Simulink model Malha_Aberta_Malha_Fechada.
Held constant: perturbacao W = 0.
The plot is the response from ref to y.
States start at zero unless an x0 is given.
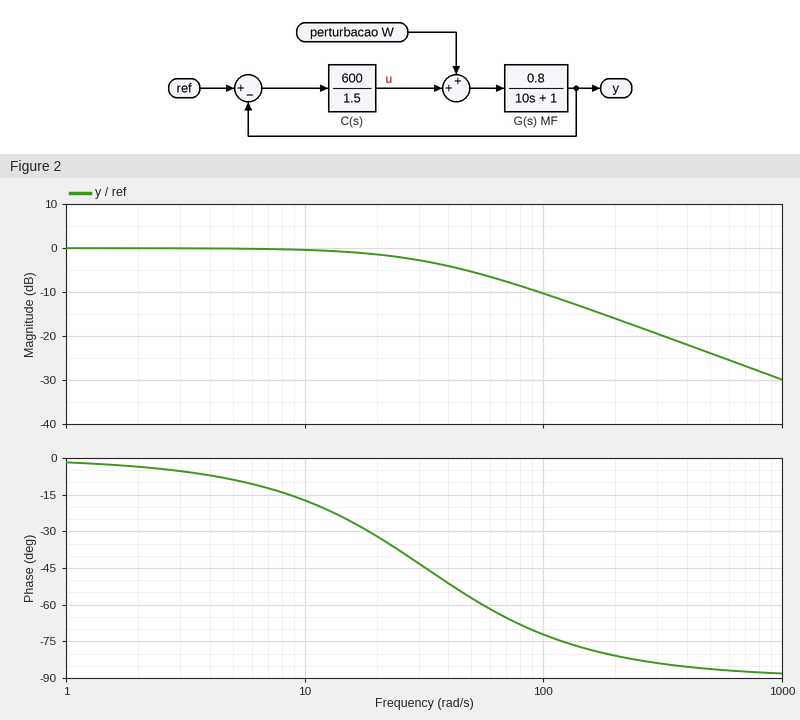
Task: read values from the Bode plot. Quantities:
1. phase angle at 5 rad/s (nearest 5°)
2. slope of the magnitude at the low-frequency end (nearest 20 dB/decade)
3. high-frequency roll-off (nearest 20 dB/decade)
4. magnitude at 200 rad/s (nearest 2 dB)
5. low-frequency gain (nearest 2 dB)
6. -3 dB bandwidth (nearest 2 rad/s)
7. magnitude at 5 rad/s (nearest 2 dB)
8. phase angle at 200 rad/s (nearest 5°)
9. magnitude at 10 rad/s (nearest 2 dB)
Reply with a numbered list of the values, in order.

1. -10°
2. 0 dB/decade
3. -20 dB/decade
4. -16 dB
5. 0 dB
6. 32 rad/s
7. 0 dB
8. -80°
9. 0 dB
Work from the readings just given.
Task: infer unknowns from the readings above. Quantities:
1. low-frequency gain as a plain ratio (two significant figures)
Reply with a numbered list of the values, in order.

1. 1.0
